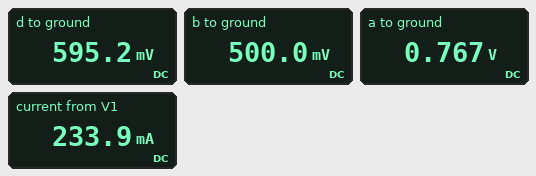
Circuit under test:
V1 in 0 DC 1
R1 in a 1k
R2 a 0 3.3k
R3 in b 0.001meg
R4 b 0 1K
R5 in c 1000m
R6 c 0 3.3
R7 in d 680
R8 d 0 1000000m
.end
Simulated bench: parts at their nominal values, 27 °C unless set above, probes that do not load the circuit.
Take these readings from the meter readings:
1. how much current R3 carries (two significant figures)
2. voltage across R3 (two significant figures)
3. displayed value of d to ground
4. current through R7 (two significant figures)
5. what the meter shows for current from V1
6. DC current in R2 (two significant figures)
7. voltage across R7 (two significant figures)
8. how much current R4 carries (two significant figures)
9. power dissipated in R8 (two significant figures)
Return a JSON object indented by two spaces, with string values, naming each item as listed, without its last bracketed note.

{
  "how much current R3 carries": "500 µA",
  "voltage across R3": "500 mV",
  "displayed value of d to ground": "595.2 mV",
  "current through R7": "600 µA",
  "what the meter shows for current from V1": "233.9 mA",
  "DC current in R2": "230 µA",
  "voltage across R7": "400 mV",
  "how much current R4 carries": "500 µA",
  "power dissipated in R8": "350 µW"
}
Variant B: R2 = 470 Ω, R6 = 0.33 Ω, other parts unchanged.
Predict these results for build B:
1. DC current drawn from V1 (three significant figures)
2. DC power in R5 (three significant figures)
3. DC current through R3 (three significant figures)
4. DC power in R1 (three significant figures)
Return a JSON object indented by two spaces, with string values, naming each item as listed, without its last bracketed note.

{
  "DC current drawn from V1": "754 mA",
  "DC power in R5": "565 mW",
  "DC current through R3": "500 µA",
  "DC power in R1": "463 µW"
}
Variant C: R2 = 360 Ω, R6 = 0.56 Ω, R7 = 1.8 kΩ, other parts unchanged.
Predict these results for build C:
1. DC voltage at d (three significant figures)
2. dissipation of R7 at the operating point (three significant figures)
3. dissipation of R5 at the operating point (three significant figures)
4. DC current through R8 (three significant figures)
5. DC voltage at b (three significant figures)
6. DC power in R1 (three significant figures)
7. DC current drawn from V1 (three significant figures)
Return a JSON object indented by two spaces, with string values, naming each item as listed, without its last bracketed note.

{
  "DC voltage at d": "357 mV",
  "dissipation of R7 at the operating point": "230 µW",
  "dissipation of R5 at the operating point": "411 mW",
  "DC current through R8": "357 µA",
  "DC voltage at b": "500 mV",
  "DC power in R1": "541 µW",
  "DC current drawn from V1": "643 mA"
}
